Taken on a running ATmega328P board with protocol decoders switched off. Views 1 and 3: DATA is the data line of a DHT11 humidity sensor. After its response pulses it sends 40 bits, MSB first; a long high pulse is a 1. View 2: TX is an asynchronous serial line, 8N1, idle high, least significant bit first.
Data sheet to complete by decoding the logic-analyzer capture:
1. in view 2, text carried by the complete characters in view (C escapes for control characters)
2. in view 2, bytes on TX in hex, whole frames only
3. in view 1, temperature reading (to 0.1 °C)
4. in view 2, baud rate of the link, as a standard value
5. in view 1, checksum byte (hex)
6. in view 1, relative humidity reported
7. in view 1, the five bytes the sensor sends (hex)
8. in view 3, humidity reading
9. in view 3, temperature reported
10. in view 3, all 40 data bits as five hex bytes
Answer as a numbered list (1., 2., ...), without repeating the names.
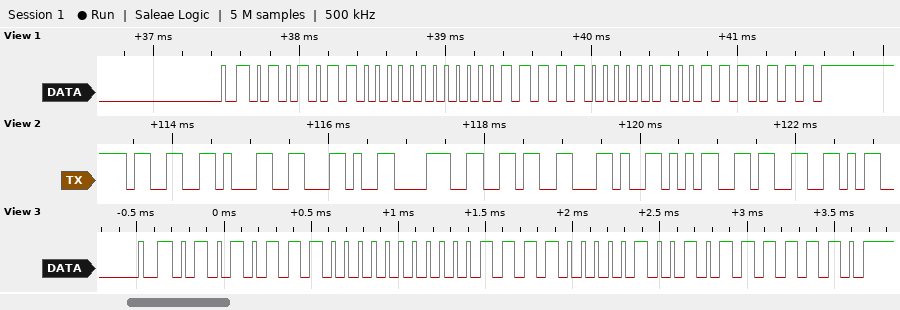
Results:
1. "31,86,53"
2. 0x33 0x31 0x2C 0x38 0x36 0x2C 0x35 0x33
3. 31.2 °C
4. 9600 baud
5. 0x77
6. 86 %
7. 56 00 1F 02 77
8. 87 %
9. 30.9 °C
10. 57 00 1E 09 7E
